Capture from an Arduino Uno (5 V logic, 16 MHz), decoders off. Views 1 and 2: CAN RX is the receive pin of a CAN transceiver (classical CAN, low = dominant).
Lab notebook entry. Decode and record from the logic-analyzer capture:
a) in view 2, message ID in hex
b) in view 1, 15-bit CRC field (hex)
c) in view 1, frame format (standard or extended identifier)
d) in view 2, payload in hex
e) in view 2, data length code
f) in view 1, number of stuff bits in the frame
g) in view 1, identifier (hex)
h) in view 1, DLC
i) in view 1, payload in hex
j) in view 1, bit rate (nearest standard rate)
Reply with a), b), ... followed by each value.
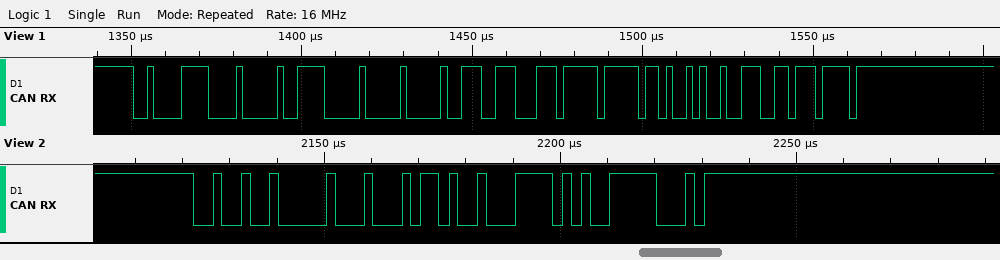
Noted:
a) 0x248
b) 0x7377
c) standard
d) 2D 23
e) 2
f) 6
g) 0x21E
h) 8
i) 0F 00 00 73 8E FF F4 A4
j) 500 kbit/s
